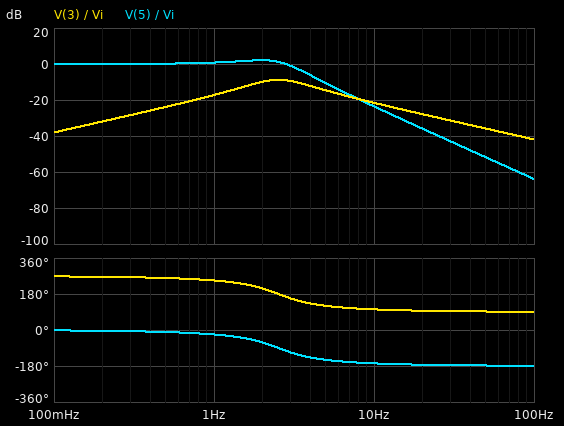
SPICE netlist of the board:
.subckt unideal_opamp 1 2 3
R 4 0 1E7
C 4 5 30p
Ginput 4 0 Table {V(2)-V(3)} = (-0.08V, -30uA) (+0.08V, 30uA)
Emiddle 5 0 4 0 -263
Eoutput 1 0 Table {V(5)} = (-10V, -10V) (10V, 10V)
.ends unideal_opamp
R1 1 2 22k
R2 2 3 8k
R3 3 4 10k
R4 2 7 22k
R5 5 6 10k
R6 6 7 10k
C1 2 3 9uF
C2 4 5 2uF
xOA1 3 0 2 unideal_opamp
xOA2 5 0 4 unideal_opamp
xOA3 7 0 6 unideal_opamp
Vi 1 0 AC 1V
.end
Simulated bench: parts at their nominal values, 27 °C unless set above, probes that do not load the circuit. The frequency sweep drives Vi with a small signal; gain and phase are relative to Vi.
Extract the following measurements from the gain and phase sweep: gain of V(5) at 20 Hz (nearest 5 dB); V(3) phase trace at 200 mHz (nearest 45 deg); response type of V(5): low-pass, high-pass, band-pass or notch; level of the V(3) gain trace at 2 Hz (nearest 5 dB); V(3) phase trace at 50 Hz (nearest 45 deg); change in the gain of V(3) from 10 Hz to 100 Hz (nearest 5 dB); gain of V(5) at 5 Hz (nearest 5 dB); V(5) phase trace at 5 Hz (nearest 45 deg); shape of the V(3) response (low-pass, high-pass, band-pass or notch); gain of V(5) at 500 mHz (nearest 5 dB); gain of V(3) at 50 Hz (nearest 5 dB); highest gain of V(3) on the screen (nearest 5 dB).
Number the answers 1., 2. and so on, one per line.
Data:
1. -35 dB
2. 270 deg
3. low-pass
4. -10 dB
5. 90 deg
6. -20 dB
7. -10 dB
8. -135 deg
9. band-pass
10. 0 dB
11. -35 dB
12. -10 dB
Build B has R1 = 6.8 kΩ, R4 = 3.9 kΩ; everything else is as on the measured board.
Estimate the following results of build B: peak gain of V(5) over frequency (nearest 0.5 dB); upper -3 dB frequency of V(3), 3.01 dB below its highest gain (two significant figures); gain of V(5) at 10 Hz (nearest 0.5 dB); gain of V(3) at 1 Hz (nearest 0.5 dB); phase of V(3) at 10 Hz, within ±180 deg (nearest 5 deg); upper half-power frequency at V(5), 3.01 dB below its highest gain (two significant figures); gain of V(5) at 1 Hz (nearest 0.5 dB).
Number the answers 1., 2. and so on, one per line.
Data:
1. 4.0 dB
2. 7.2 Hz
3. -10.5 dB
4. -22.5 dB
5. 110 deg
6. 6.8 Hz
7. -4.5 dB
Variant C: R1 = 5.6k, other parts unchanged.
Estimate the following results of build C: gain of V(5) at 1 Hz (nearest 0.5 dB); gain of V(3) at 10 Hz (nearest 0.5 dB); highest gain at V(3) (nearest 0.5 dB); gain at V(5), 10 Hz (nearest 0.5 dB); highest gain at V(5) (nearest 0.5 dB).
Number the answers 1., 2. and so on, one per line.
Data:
1. 12.5 dB
2. -9.5 dB
3. 3.0 dB
4. -11.5 dB
5. 14.0 dB
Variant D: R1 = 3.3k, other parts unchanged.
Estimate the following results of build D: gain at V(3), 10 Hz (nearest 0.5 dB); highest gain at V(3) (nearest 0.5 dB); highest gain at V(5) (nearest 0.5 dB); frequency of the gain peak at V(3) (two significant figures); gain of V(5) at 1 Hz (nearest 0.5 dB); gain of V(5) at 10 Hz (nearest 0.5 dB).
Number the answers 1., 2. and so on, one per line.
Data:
1. -5.0 dB
2. 7.5 dB
3. 18.5 dB
4. 2.5 Hz
5. 17.5 dB
6. -7.0 dB
